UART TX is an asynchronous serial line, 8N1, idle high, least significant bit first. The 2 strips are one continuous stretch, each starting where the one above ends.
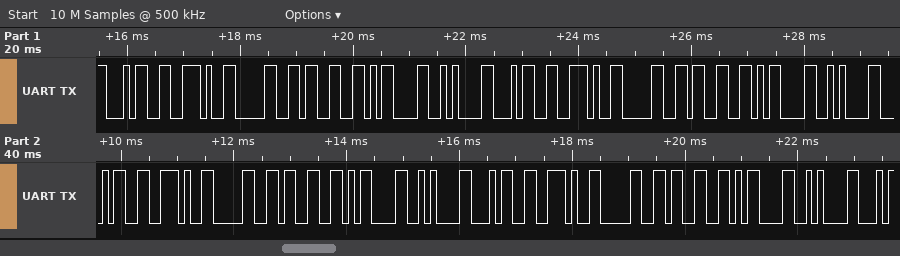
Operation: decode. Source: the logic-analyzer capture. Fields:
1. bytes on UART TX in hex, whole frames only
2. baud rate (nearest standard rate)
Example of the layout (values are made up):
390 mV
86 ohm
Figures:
34 2E 30 33 0D 0A 34 2E 30 33 0D 0A 34 2E 30 33 0D 0A 34 2E 30 33 0D 0A
9600 baud
